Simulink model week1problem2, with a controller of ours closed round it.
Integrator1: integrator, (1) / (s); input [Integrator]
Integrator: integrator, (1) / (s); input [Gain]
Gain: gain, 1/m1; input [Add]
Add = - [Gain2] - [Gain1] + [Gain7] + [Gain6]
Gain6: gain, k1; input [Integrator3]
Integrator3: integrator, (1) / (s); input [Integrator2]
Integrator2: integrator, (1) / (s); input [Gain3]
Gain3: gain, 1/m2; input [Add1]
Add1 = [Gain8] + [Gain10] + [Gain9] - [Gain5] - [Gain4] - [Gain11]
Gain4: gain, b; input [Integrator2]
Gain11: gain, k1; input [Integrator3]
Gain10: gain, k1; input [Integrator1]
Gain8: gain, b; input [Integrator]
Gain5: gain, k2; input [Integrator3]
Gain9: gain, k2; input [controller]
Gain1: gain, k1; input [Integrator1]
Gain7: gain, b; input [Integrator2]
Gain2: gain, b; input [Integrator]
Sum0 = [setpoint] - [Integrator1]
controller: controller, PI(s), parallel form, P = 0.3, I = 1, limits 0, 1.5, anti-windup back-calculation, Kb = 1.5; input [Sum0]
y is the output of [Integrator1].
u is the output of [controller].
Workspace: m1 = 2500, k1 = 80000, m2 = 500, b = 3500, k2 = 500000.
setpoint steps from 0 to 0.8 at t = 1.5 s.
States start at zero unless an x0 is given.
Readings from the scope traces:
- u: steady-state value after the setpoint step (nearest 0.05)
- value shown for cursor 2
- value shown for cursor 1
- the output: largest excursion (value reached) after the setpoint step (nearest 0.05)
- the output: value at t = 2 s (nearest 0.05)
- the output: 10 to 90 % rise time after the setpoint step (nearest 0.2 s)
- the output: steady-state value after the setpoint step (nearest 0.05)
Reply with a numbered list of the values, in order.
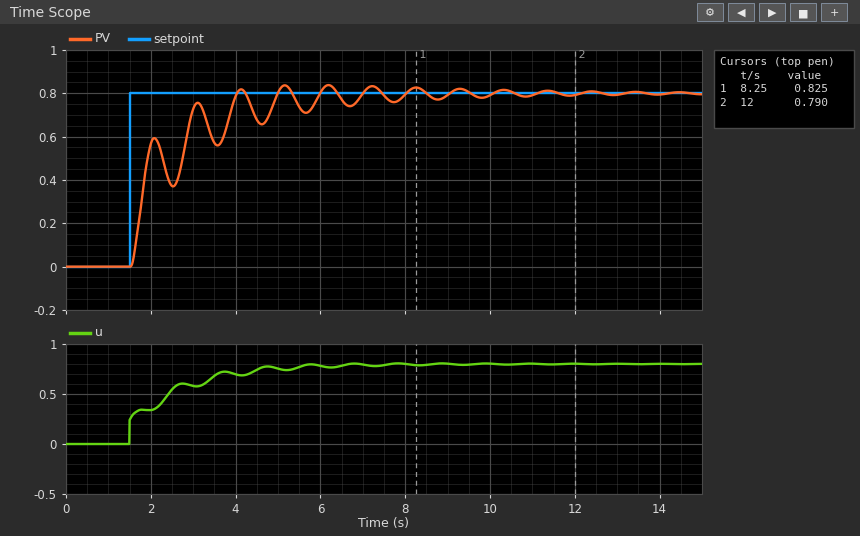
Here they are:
1. 0.80
2. 0.790
3. 0.825
4. 0.85
5. 0.55
6. 1.4 s
7. 0.80
